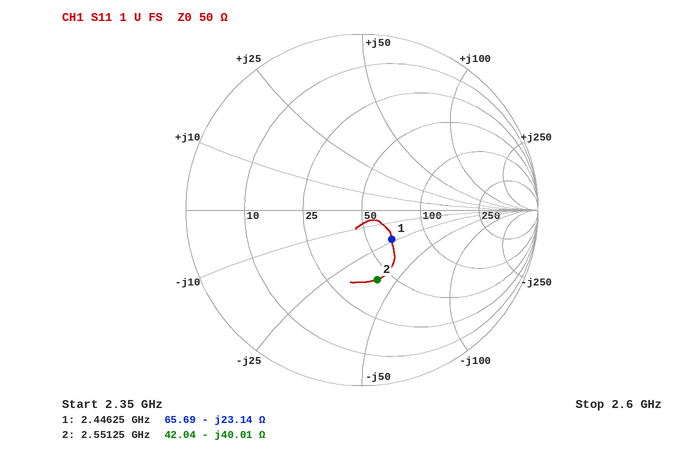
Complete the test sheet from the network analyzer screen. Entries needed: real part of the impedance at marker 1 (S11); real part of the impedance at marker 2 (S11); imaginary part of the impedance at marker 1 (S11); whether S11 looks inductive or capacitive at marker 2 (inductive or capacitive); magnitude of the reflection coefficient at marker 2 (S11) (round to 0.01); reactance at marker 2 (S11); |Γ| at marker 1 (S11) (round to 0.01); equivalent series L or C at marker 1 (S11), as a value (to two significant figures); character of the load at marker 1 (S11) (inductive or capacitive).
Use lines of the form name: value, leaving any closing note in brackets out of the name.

real part of the impedance at marker 1: 65.69 Ω
real part of the impedance at marker 2: 42.04 Ω
imaginary part of the impedance at marker 1: -23.14 Ω
whether S11 looks inductive or capacitive at marker 2: capacitive
magnitude of the reflection coefficient at marker 2 (S11): 0.41
reactance at marker 2: -40.01 Ω
|Γ| at marker 1 (S11): 0.24
equivalent series L or C at marker 1 (S11), as a value: 2.8 pF
character of the load at marker 1 (S11): capacitive
